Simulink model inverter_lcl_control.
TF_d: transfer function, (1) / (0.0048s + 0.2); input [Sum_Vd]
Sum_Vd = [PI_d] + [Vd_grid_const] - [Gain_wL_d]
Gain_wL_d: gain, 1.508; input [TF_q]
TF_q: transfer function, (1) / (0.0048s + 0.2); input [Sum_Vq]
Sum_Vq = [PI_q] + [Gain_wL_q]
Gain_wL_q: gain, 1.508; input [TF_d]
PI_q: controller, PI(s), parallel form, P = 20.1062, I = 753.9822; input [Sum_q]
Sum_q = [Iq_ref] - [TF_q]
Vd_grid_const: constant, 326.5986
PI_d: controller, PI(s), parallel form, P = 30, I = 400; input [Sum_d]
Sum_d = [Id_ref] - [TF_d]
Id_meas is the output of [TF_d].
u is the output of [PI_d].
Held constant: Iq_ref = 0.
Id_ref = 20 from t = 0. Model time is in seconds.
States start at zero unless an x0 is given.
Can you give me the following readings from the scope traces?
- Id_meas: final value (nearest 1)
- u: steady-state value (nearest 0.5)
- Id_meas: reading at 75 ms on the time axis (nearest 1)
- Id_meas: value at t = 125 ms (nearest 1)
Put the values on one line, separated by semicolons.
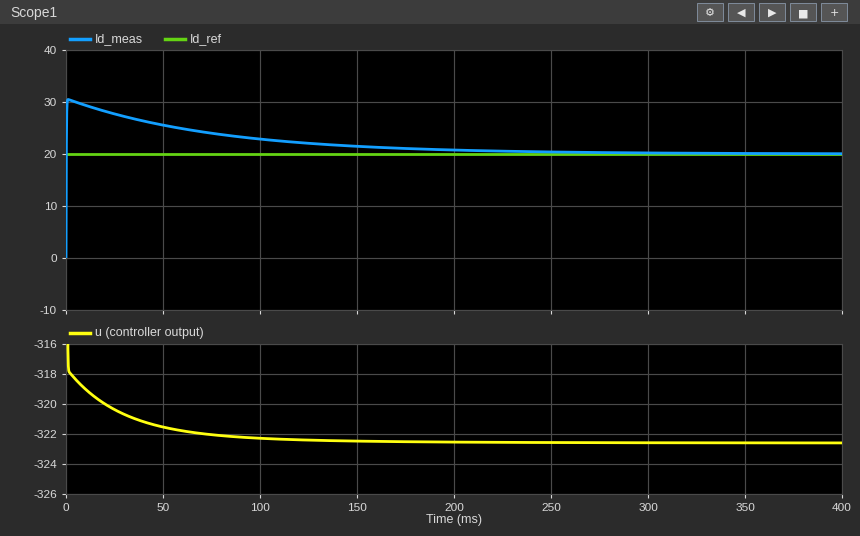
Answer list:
20; -322.5; 24; 22
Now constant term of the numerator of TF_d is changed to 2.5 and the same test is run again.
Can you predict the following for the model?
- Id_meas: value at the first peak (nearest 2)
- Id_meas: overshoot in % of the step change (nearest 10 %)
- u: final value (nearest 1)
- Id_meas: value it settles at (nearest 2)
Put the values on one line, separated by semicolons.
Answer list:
30; 50 %; -325; 20
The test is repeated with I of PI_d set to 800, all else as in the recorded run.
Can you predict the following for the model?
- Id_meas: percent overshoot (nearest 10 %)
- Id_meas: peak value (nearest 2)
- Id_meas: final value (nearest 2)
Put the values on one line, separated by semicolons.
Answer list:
50 %; 30; 20
